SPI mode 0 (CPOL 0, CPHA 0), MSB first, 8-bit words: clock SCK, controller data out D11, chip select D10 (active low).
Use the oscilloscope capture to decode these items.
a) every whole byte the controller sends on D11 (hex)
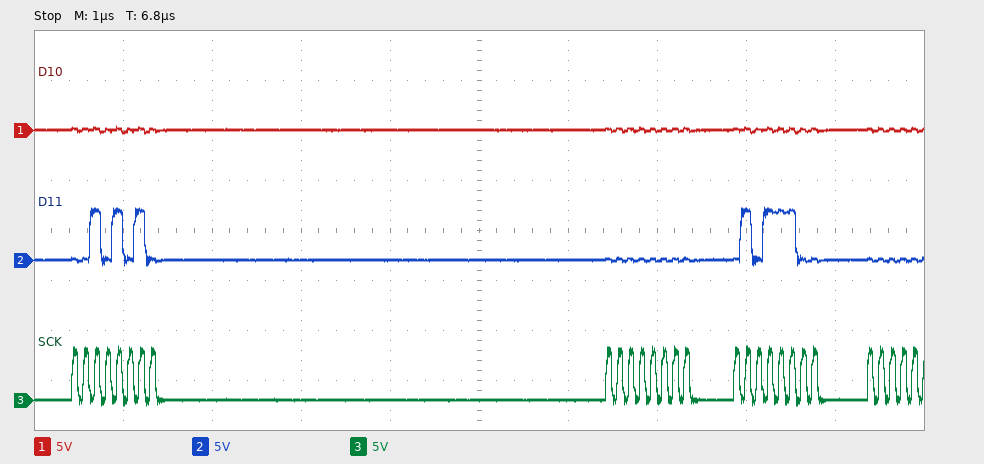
2A 00 5C
